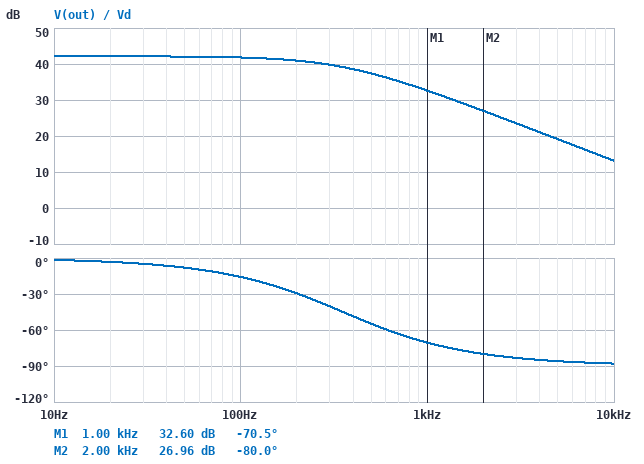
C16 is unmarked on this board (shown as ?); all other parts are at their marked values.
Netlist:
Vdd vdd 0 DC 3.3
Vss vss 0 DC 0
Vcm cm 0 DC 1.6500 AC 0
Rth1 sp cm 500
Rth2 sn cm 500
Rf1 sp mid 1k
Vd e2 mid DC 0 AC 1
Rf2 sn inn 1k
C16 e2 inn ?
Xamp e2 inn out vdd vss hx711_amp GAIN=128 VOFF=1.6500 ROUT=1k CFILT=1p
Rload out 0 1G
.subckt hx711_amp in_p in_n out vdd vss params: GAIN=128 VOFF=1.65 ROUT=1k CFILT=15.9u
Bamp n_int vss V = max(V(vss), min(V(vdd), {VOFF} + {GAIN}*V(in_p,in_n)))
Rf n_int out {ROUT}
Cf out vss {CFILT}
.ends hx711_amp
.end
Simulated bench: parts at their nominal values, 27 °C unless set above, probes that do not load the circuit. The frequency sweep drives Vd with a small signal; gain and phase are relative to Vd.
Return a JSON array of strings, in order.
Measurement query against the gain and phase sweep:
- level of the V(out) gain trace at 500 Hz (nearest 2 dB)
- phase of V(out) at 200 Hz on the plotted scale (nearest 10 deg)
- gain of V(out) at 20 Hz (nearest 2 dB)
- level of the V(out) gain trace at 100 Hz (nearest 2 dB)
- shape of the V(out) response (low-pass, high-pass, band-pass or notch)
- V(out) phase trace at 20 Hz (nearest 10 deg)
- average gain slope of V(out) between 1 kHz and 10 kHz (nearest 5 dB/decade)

["38 dB", "-30 deg", "42 dB", "42 dB", "low-pass", "0 deg", "-20 dB/decade"]
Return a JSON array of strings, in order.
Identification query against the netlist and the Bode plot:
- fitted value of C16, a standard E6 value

["150 nF"]
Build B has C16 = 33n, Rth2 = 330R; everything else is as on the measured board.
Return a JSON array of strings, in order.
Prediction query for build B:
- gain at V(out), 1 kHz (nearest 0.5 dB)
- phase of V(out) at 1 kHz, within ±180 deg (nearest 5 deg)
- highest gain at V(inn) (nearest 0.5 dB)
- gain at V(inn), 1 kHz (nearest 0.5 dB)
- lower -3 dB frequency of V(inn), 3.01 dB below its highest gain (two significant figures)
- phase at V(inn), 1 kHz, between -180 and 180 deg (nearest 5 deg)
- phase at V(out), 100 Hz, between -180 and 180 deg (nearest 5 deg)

["41.0 dB", "-30 deg", "-6.5 dB", "-12.5 dB", "1.7 kHz", "60 deg", "-5 deg"]
